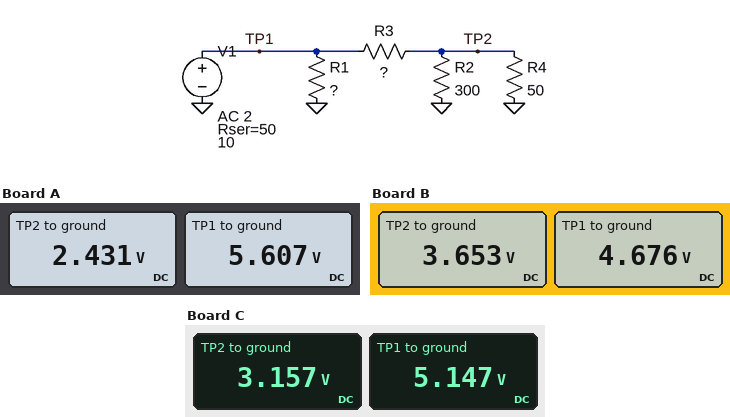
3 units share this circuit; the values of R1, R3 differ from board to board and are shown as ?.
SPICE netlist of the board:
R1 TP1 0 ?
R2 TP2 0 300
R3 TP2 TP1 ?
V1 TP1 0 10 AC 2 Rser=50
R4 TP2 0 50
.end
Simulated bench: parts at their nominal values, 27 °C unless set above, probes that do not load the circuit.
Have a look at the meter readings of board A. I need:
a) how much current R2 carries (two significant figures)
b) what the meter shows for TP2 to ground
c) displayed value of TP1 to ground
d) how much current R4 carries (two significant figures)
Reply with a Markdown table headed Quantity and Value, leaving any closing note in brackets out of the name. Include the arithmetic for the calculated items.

| Quantity | Value |
|---|---|
| how much current R2 carries | (2.431 V) / 300 Ω = 8.1 mA |
| what the meter shows for TP2 to ground | 2.431 V |
| displayed value of TP1 to ground | 5.607 V |
| how much current R4 carries | (2.431 V) / 50 Ω = 49 mA |
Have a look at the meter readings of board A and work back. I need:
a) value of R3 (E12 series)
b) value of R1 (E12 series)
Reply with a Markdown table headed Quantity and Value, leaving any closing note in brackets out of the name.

| Quantity | Value |
|---|---|
| value of R3 | 56 Ω |
| value of R1 | 180 Ω |
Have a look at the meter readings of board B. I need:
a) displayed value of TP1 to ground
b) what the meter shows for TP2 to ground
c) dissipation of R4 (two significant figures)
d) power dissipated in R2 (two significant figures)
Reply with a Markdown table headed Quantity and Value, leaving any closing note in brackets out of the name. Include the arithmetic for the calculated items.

| Quantity | Value |
|---|---|
| displayed value of TP1 to ground | 4.676 V |
| what the meter shows for TP2 to ground | 3.653 V |
| dissipation of R4 | (3.653 V)^2 / 50 Ω = 270 mW |
| power dissipated in R2 | (3.653 V)^2 / 300 Ω = 44 mW |
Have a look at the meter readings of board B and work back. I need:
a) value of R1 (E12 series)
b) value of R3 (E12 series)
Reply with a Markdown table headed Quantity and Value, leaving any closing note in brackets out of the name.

| Quantity | Value |
|---|---|
| value of R1 | 220 Ω |
| value of R3 | 12 Ω |
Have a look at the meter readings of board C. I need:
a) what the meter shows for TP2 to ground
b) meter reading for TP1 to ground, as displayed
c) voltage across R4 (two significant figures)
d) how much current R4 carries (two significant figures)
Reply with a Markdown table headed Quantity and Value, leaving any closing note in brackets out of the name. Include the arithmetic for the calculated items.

| Quantity | Value |
|---|---|
| what the meter shows for TP2 to ground | 3.157 V |
| meter reading for TP1 to ground, as displayed | 5.147 V |
| voltage across R4 | 3.157 V = 3.2 V |
| how much current R4 carries | (3.157 V) / 50 Ω = 63 mA |
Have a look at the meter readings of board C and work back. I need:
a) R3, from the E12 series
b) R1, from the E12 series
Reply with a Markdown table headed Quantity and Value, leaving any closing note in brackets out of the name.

| Quantity | Value |
|---|---|
| R3, from the E12 series | 27 Ω |
| R1, from the E12 series | 220 Ω |
